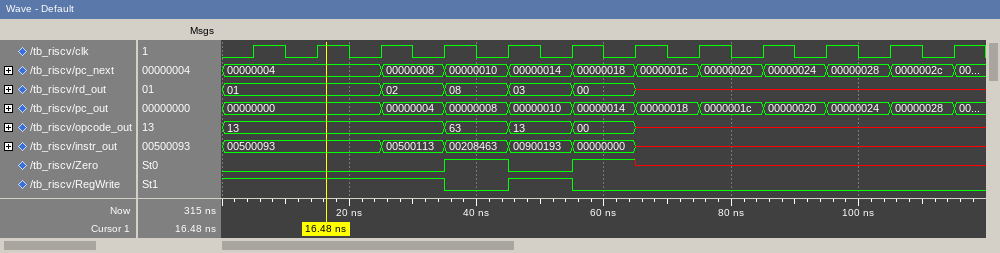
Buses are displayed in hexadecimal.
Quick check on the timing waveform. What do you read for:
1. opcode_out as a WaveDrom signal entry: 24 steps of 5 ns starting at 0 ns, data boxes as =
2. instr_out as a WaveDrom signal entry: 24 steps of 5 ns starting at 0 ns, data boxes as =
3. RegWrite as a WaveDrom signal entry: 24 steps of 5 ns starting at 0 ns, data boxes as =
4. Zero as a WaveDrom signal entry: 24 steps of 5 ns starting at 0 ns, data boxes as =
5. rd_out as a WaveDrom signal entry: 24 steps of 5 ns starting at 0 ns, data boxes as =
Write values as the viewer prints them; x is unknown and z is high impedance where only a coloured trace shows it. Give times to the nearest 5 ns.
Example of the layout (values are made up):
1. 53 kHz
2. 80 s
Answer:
1. {name: 'opcode_out', wave: '=......=.=.=.x..........', data: '13 63 13 00'}
2. {name: 'instr_out', wave: '=....=.=.=.=.x..........', data: '00500093 00500113 00208463 00900193 00000000'}
3. {name: 'RegWrite', wave: '1......0.1.0............'}
4. {name: 'Zero', wave: '0......1.0.1.x..........'}
5. {name: 'rd_out', wave: '=....=.=.=.=.x..........', data: '01 02 08 03 00'}
